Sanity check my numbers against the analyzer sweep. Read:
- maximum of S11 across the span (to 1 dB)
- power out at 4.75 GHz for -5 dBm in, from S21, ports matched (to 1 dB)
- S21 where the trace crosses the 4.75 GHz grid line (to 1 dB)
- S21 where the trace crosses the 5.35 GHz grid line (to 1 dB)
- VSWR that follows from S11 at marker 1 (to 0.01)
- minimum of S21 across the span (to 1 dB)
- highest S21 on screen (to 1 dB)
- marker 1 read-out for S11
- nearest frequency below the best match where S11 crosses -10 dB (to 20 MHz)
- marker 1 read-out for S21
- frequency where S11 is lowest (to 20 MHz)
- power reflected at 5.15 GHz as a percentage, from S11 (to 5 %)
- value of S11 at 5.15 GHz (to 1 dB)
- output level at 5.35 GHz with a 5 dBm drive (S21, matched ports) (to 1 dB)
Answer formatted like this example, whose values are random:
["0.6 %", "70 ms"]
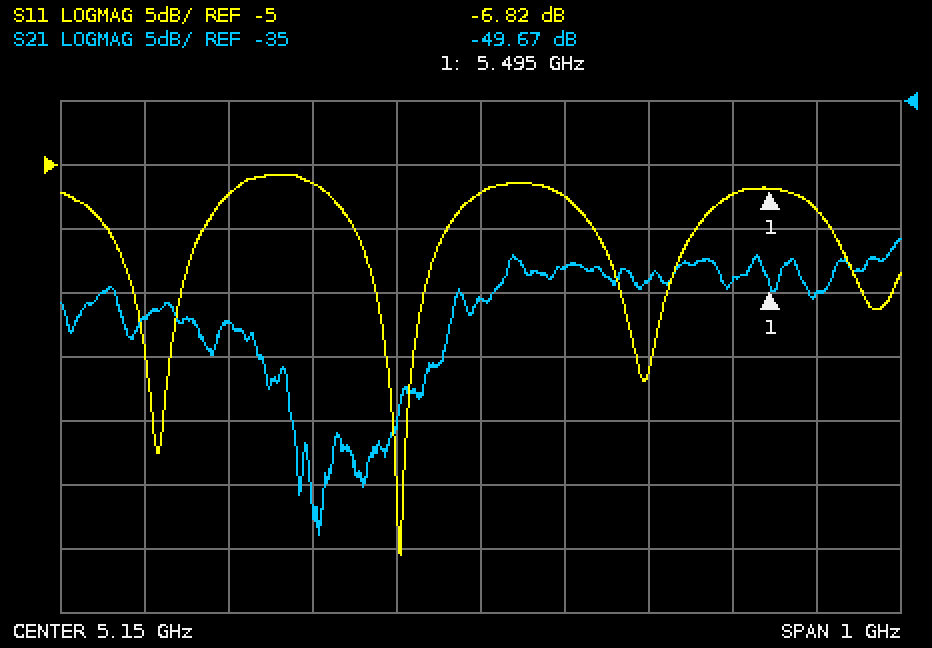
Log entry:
["-6 dB", "-57 dBm", "-52 dB", "-49 dB", "2.68", "-69 dB", "-46 dB", "-6.82 dB", "5.00 GHz", "-49.67 dB", "5.06 GHz", "20 %", "-7 dB", "-44 dBm"]
